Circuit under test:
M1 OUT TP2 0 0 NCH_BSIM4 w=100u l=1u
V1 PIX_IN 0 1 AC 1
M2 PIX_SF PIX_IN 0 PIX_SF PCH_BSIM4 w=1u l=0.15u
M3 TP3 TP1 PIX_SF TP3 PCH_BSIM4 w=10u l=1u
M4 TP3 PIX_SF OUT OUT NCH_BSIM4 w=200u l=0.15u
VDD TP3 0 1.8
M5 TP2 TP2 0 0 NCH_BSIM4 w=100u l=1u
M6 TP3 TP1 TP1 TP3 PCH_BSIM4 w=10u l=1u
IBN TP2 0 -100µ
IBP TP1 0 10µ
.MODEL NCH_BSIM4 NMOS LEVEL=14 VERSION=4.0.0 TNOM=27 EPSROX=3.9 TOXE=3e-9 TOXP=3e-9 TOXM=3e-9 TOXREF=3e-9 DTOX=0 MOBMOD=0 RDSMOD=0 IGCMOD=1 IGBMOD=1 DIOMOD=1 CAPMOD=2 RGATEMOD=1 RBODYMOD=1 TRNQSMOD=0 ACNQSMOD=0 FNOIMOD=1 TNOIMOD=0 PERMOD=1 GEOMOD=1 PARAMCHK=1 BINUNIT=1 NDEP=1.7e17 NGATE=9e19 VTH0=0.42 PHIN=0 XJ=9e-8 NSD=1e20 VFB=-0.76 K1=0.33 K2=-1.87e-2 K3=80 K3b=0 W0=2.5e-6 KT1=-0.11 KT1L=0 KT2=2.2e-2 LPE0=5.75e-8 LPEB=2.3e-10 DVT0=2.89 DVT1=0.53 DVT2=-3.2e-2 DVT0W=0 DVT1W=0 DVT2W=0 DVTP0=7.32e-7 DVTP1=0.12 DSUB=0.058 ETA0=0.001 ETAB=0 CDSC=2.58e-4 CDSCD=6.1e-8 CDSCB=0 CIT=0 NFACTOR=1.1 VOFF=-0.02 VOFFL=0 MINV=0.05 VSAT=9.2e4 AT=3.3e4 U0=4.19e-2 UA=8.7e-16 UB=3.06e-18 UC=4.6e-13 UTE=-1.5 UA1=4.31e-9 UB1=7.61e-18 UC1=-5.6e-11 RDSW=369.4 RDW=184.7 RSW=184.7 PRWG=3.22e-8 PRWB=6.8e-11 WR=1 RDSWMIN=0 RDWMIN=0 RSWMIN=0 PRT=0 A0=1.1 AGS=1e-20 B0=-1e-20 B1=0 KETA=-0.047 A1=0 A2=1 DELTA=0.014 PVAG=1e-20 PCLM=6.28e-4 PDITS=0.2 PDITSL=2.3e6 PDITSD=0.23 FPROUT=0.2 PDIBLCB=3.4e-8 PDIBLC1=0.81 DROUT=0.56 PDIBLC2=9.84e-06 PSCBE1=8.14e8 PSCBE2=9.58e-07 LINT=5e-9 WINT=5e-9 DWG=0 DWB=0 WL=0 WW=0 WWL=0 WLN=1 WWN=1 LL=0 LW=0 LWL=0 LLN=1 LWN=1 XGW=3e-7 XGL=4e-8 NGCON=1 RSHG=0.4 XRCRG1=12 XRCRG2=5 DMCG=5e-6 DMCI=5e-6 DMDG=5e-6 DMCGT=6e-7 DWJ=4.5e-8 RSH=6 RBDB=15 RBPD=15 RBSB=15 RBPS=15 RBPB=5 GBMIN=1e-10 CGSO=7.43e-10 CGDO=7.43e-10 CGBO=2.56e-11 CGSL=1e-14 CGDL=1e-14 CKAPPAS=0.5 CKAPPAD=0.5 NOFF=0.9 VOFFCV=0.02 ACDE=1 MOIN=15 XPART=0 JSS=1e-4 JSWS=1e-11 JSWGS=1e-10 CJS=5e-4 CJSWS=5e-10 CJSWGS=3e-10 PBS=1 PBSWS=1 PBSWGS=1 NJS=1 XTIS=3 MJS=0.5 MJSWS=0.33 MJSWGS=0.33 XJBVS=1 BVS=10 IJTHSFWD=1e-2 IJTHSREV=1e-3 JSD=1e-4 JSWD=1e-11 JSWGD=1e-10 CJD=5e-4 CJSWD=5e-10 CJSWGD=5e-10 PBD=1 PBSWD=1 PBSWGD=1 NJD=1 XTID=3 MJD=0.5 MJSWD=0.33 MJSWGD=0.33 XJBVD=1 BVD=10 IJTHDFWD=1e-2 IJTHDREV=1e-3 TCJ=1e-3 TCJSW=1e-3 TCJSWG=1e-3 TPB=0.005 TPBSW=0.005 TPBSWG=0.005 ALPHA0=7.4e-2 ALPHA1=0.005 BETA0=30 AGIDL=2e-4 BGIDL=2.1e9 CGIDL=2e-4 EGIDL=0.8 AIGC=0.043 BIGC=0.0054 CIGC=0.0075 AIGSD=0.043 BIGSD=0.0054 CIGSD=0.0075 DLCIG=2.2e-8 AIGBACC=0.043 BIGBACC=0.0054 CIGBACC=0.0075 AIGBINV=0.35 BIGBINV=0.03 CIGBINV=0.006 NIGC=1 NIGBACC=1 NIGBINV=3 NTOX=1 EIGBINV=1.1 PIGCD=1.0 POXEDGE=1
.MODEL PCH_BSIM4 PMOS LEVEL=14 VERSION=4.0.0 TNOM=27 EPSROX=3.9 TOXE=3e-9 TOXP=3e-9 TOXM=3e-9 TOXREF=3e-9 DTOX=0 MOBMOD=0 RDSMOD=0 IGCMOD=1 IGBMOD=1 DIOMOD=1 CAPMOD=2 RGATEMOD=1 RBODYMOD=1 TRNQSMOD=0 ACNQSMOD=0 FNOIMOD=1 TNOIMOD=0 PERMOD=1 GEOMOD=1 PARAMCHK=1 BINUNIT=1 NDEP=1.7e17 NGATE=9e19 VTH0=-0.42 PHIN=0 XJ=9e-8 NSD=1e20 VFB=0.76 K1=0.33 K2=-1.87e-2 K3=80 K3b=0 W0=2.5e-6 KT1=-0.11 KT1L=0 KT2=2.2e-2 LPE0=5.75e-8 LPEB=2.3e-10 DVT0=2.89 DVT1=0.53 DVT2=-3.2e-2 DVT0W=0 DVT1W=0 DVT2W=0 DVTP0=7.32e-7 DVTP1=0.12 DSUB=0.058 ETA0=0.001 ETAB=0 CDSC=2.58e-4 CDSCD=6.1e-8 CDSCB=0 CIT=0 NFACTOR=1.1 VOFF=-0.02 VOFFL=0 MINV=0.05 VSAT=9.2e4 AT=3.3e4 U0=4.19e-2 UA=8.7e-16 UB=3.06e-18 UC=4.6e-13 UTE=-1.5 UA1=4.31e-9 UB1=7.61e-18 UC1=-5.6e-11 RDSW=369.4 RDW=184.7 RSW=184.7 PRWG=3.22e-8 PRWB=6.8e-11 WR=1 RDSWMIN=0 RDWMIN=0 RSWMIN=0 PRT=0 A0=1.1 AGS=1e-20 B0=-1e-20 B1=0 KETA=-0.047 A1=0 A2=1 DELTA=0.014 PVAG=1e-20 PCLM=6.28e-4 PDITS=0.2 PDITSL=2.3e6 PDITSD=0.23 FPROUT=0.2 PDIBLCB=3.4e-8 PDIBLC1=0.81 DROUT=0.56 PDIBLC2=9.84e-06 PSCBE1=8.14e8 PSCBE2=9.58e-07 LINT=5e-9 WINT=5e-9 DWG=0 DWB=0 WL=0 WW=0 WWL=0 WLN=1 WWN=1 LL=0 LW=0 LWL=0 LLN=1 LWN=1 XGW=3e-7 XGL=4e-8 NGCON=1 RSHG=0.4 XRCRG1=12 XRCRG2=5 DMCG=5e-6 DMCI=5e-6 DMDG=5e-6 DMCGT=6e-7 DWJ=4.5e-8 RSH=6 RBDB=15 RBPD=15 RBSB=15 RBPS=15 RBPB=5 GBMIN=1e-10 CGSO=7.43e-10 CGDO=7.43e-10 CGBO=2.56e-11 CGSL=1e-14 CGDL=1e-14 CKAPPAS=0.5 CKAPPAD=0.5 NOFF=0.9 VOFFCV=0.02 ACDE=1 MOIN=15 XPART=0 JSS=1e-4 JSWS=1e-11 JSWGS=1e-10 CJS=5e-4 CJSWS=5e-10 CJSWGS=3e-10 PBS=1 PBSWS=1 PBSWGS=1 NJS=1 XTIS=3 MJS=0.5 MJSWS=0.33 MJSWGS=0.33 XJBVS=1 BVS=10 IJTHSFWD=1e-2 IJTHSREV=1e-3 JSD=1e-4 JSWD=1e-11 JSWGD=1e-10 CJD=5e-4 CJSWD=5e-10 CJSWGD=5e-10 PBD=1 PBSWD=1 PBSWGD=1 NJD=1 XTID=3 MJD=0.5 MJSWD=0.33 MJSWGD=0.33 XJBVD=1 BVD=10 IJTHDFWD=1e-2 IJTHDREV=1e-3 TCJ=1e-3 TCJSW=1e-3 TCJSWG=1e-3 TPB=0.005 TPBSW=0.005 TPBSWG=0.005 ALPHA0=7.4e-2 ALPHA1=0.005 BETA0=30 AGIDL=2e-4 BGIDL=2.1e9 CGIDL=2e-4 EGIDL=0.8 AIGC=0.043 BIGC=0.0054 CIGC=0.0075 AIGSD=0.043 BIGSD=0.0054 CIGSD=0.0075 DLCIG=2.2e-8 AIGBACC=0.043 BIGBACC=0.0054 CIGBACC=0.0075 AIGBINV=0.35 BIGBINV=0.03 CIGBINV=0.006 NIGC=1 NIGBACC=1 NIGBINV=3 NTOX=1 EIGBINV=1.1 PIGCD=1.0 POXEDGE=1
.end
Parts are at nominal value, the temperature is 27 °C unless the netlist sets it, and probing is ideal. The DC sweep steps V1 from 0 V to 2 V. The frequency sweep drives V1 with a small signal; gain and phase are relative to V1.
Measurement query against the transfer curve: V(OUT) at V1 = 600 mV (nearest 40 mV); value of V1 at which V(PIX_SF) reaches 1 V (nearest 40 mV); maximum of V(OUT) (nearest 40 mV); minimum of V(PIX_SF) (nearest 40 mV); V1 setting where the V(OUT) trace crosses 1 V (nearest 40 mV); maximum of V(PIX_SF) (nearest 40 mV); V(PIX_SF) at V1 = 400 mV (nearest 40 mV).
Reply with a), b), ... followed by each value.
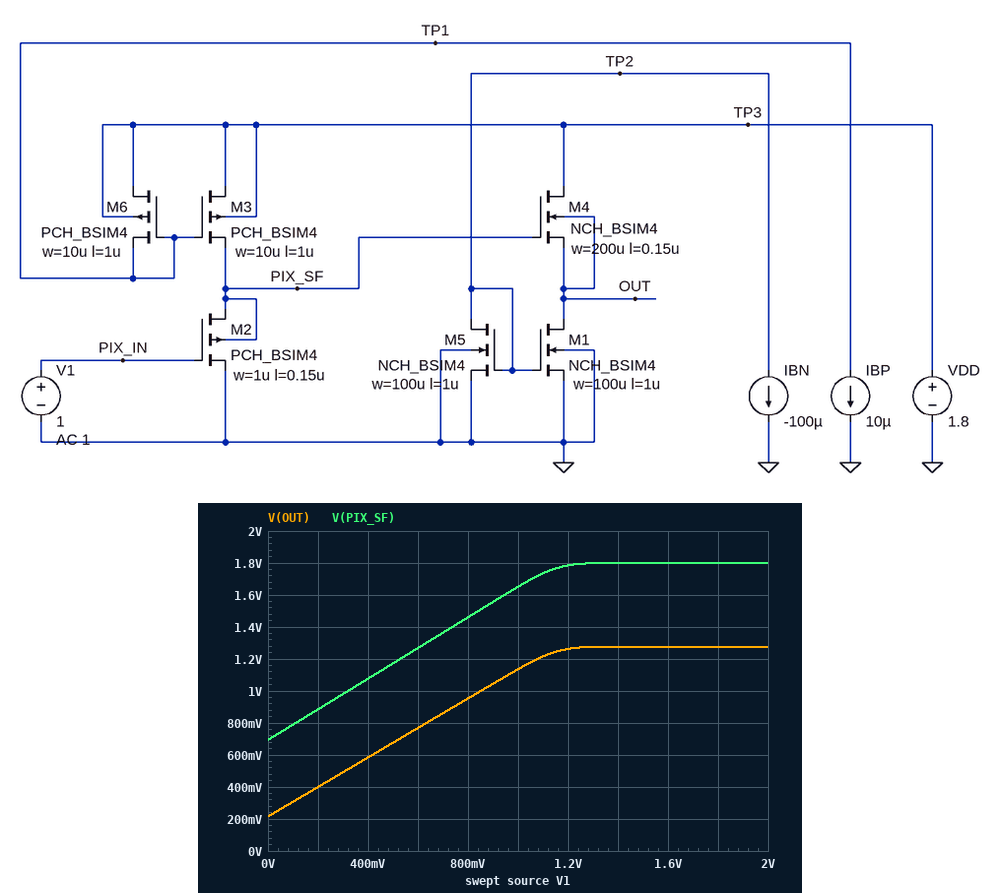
a) 760 mV
b) 320 mV
c) 1.28 V
d) 680 mV
e) 840 mV
f) 1.80 V
g) 1.08 V
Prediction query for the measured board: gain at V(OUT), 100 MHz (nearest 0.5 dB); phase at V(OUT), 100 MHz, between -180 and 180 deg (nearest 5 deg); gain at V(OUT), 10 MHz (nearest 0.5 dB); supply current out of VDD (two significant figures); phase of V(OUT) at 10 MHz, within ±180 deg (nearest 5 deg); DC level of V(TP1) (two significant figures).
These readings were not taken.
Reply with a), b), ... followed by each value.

a) -3.5 dB
b) -55 deg
c) -1.0 dB
d) 120 µA
e) -5 deg
f) 1.2 V
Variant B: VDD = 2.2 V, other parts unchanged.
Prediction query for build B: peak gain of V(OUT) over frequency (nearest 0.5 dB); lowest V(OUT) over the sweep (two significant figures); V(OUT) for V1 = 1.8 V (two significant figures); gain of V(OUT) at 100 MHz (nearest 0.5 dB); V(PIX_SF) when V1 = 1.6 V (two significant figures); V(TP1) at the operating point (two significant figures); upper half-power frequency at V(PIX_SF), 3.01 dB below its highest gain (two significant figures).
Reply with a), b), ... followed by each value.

a) -0.5 dB
b) 230 mV
c) 1.7 V
d) -3.0 dB
e) 2.2 V
f) 1.6 V
g) 130 MHz
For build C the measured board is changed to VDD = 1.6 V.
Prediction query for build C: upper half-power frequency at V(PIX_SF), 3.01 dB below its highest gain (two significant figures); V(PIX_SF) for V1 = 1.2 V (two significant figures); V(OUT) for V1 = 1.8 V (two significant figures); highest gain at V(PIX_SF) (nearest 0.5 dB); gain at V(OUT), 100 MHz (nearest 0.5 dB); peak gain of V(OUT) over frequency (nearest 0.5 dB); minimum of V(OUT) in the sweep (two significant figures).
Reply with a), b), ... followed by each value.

a) 110 MHz
b) 1.6 V
c) 1.1 V
d) -11.5 dB
e) -15.0 dB
f) -12.0 dB
g) 210 mV
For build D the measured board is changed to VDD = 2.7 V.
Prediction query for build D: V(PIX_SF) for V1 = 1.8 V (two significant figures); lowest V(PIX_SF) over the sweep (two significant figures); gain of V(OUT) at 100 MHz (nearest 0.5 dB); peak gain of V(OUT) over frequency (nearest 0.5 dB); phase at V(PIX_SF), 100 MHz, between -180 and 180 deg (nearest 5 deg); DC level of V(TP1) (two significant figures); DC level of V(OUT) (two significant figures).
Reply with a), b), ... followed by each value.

a) 2.4 V
b) 700 mV
c) -2.5 dB
d) -0.5 dB
e) -40 deg
f) 2.1 V
g) 1.2 V
